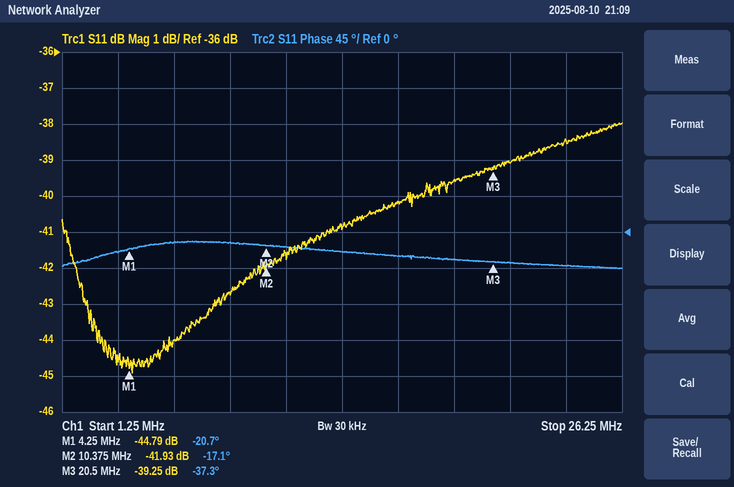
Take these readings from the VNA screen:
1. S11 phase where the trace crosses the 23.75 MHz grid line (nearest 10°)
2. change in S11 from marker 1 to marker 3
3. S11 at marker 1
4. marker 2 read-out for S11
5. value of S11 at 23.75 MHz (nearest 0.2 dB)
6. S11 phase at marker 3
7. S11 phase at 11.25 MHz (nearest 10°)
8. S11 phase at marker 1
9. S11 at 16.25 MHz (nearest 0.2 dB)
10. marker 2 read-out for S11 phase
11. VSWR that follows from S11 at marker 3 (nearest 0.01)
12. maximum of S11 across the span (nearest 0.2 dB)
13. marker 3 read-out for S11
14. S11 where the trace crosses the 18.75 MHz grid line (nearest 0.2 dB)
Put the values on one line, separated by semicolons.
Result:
-40°; 5.54 dB; -44.79 dB; -41.93 dB; -38.4 dB; -37.3°; -20°; -20.7°; -40.2 dB; -17.1°; 1.02; -38.0 dB; -39.25 dB; -39.6 dB
